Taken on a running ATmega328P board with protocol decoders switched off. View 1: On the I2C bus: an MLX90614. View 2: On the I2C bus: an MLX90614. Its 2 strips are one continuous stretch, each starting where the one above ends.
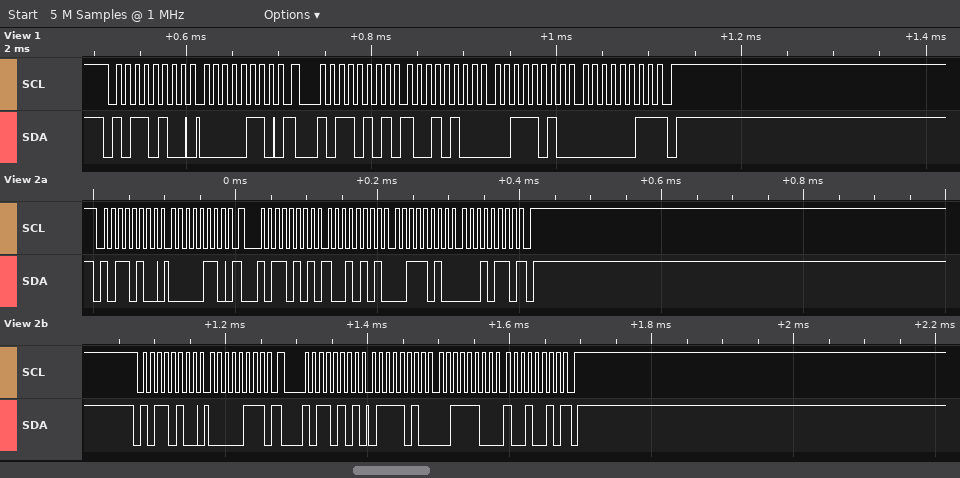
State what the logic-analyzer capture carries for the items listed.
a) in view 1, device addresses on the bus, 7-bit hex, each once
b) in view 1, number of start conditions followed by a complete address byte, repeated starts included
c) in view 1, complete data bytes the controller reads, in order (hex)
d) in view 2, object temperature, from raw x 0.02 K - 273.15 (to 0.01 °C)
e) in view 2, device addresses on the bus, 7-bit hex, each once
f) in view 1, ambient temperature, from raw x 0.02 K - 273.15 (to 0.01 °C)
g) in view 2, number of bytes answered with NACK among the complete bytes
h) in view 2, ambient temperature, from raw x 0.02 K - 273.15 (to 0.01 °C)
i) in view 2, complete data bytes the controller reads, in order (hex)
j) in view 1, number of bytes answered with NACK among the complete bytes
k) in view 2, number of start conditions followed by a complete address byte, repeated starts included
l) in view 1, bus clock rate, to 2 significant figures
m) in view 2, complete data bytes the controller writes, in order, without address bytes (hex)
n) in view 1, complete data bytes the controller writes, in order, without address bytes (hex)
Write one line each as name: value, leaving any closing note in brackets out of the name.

in view 1, device addresses on the bus, 7-bit hex, each once: 0x5A
in view 1, number of start conditions followed by a complete address byte, repeated starts included: 2
in view 1, complete data bytes the controller reads, in order: 94 3A 03
in view 2, object temperature, from raw x 0.02 K - 273.15: 36.49 °C
in view 2, device addresses on the bus, 7-bit hex, each once: 0x5A
in view 1, ambient temperature, from raw x 0.02 K - 273.15: 26.77 °C
in view 2, number of bytes answered with NACK among the complete bytes: 2
in view 2, ambient temperature, from raw x 0.02 K - 273.15: 26.79 °C
in view 2, complete data bytes the controller reads, in order: 95 3A 16 7A 3C 92
in view 1, number of bytes answered with NACK among the complete bytes: 1
in view 2, number of start conditions followed by a complete address byte, repeated starts included: 4
in view 1, bus clock rate, to 2 significant figures: 100 kHz
in view 2, complete data bytes the controller writes, in order, without address bytes: 06 07
in view 1, complete data bytes the controller writes, in order, without address bytes: 06
